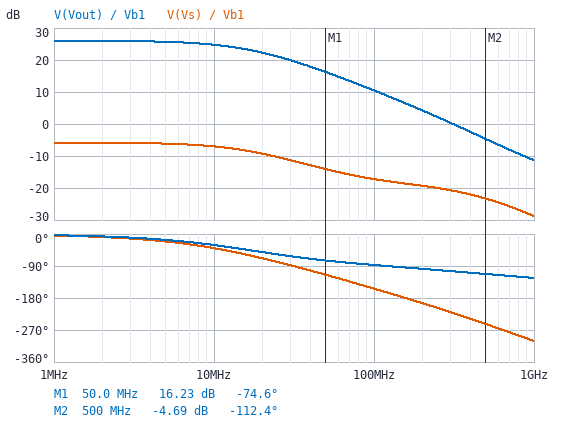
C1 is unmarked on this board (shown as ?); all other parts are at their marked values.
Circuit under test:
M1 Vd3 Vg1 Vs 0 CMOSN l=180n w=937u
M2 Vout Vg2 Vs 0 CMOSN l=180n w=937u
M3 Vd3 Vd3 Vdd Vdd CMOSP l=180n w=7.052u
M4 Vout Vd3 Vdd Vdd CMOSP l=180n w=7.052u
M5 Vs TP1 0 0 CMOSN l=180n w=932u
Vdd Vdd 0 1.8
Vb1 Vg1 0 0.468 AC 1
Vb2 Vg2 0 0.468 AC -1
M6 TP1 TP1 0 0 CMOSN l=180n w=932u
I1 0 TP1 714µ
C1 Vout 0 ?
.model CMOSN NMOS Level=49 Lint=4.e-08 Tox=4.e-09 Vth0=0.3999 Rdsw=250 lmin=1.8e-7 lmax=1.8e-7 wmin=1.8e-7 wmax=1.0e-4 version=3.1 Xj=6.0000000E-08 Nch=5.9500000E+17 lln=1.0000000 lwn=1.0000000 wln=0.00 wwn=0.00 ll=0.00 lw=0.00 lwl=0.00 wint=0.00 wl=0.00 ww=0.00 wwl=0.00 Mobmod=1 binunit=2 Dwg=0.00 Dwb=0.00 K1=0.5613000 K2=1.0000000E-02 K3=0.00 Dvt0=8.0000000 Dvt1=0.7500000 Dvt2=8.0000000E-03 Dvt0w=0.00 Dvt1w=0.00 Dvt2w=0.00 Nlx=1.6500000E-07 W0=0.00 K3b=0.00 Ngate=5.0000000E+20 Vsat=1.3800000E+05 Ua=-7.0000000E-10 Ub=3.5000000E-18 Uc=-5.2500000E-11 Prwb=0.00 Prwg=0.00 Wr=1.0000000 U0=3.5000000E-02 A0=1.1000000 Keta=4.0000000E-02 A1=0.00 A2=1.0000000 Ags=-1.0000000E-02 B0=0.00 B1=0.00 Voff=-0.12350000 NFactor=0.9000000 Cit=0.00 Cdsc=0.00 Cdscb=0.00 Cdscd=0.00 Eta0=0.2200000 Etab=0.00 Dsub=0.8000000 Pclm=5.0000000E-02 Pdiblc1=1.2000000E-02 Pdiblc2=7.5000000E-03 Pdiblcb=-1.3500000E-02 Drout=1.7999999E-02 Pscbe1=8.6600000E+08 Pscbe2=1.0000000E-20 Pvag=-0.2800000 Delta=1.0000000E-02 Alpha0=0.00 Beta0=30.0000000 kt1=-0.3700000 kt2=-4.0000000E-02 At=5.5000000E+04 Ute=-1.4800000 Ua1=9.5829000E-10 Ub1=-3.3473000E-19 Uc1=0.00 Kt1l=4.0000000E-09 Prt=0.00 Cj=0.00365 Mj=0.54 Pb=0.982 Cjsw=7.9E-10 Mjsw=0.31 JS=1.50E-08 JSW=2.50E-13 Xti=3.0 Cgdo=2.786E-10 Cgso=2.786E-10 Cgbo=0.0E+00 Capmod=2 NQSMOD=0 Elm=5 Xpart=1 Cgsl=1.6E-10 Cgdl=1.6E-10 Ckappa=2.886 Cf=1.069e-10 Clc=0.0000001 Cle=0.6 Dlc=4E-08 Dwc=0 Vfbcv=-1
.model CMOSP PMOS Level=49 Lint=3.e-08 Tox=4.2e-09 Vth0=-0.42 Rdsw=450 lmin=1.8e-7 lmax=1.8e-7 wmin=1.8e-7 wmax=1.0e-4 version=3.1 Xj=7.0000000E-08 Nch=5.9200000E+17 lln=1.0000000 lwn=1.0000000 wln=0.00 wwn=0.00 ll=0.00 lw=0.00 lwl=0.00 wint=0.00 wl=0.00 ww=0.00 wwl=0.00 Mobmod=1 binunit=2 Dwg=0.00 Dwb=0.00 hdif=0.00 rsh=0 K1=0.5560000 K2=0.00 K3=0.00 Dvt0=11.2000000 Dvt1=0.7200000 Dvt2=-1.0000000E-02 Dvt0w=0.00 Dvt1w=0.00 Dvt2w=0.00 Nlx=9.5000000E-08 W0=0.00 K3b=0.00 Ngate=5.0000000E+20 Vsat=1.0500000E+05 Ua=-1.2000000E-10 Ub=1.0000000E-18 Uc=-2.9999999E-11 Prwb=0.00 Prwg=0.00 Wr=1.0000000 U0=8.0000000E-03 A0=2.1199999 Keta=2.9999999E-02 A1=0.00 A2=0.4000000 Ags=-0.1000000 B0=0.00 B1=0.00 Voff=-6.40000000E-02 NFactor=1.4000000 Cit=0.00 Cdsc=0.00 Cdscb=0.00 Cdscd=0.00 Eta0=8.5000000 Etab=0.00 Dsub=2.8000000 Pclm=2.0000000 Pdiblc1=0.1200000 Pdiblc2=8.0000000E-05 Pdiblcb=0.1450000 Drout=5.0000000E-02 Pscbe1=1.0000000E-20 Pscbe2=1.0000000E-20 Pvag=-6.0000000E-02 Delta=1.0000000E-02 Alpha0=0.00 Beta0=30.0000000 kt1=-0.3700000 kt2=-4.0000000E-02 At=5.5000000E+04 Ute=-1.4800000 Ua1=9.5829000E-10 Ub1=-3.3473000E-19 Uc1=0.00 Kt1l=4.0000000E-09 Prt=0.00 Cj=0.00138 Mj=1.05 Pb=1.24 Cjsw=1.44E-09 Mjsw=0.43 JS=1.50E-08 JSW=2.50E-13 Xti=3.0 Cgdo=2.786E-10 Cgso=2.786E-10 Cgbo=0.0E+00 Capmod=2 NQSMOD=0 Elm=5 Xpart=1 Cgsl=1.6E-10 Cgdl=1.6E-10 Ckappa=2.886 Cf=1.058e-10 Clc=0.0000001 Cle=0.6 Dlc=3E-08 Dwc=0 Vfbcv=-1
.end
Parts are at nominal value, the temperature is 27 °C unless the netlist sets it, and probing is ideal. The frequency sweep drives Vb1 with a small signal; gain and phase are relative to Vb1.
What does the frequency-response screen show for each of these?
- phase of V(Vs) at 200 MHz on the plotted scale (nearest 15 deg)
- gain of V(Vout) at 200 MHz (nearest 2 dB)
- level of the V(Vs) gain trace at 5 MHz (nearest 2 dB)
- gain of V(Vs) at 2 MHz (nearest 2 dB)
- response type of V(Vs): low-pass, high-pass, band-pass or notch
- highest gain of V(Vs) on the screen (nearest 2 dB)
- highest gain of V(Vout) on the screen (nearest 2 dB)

-195 deg
4 dB
-6 dB
-6 dB
low-pass
-6 dB
26 dB
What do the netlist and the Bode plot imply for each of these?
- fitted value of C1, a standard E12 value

3.9 pF
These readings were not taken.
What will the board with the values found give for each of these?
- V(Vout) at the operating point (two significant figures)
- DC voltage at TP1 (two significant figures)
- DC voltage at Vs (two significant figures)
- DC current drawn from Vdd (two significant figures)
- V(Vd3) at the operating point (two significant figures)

1.1 V
340 mV
190 mV
530 µA
1.1 V
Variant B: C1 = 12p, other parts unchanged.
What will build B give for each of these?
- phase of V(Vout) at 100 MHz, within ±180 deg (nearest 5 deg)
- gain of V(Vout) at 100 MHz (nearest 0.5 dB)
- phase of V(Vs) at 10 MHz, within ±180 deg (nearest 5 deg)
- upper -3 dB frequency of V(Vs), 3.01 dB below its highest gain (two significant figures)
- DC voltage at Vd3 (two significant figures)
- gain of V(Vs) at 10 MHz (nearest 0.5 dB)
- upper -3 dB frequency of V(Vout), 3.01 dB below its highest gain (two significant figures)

-95 deg
2.0 dB
-80 deg
6.9 MHz
1.1 V
-10.5 dB
6.5 MHz
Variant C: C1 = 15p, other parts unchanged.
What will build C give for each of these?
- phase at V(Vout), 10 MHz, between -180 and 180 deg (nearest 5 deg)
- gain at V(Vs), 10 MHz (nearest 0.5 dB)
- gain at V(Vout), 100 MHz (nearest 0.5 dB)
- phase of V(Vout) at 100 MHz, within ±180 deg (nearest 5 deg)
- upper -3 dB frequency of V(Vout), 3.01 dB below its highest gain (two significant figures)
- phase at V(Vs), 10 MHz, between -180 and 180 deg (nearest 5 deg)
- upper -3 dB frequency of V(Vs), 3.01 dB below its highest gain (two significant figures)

-65 deg
-11.5 dB
0.5 dB
-95 deg
5.3 MHz
-90 deg
5.6 MHz
